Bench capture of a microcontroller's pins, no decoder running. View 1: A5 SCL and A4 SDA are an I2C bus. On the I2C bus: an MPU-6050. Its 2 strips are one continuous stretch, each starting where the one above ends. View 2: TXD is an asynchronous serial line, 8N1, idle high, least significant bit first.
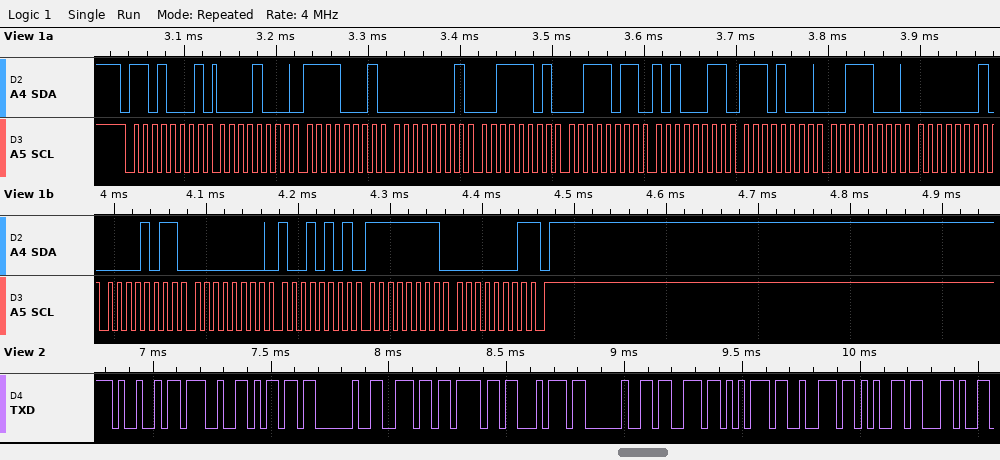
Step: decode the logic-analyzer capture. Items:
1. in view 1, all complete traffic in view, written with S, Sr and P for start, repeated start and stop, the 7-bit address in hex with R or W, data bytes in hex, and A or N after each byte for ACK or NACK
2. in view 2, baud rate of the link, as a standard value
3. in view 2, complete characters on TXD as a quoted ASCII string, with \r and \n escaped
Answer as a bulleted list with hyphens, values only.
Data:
- S 68R A 08 A F1 A 01 A 3D A 3B A A3 A E8 A 38 A 01 A 0B A 00 A 95 A FF A 01 N P
- 38400 baud
- "I'm not sure,"
